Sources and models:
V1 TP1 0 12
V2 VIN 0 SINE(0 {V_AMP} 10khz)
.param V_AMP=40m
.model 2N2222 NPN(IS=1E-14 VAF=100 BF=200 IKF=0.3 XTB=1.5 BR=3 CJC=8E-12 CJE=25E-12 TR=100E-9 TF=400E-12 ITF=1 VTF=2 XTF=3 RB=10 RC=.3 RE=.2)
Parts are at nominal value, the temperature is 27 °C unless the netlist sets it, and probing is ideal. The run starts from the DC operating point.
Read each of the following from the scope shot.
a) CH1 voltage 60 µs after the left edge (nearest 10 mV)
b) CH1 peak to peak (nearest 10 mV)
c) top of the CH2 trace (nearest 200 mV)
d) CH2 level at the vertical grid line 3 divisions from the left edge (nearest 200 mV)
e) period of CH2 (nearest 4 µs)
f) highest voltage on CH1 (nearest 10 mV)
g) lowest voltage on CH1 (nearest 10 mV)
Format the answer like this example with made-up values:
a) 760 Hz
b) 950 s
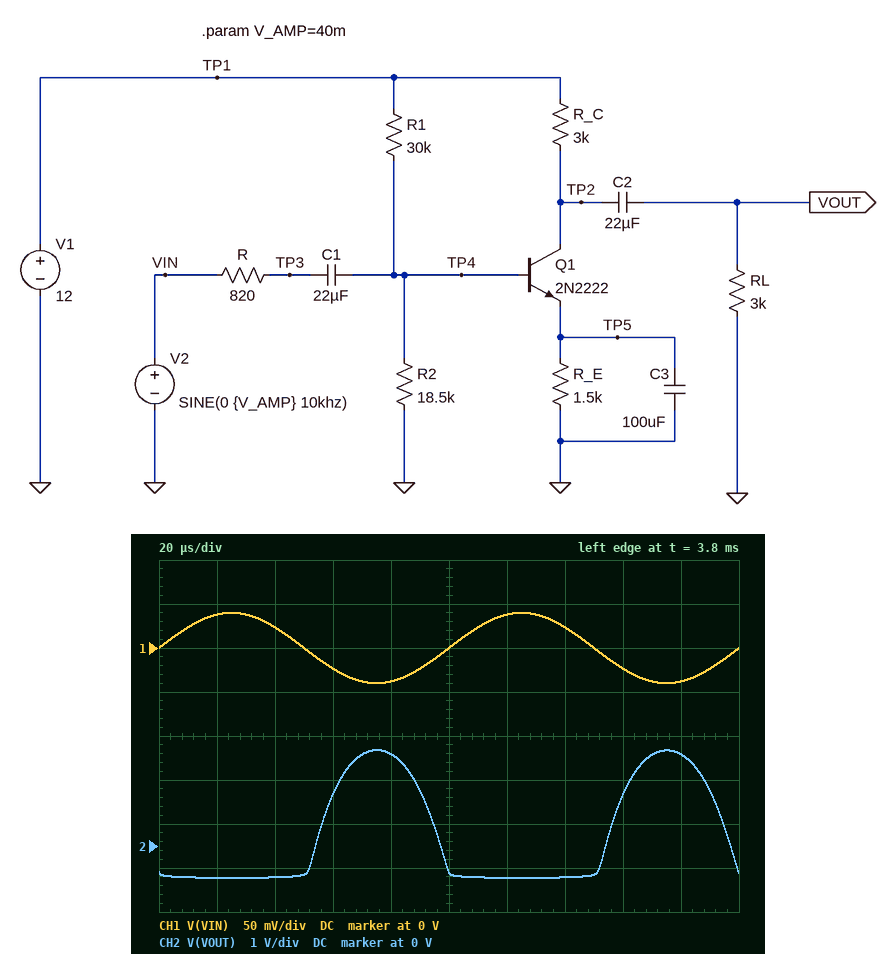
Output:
a) -20 mV
b) 80 mV
c) 2.2 V
d) 1.2 V
e) 100 µs
f) 40 mV
g) -40 mV
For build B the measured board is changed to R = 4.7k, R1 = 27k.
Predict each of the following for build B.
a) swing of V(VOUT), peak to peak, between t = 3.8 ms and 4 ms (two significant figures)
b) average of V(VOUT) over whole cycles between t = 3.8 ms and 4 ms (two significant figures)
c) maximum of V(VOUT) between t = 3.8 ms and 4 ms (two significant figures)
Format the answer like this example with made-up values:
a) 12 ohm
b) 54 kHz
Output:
a) 260 mV
b) 30 mV
c) 240 mV
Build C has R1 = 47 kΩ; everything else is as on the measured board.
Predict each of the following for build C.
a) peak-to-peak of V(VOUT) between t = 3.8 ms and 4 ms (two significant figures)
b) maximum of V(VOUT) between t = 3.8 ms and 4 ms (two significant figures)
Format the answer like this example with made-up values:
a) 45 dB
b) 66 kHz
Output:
a) 5.2 V
b) 2.0 V
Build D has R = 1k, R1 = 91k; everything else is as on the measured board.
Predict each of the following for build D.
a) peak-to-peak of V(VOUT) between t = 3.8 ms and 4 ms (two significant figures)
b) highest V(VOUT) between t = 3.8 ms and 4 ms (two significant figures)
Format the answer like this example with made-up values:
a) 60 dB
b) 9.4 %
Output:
a) 3.1 V
b) 1.0 V
